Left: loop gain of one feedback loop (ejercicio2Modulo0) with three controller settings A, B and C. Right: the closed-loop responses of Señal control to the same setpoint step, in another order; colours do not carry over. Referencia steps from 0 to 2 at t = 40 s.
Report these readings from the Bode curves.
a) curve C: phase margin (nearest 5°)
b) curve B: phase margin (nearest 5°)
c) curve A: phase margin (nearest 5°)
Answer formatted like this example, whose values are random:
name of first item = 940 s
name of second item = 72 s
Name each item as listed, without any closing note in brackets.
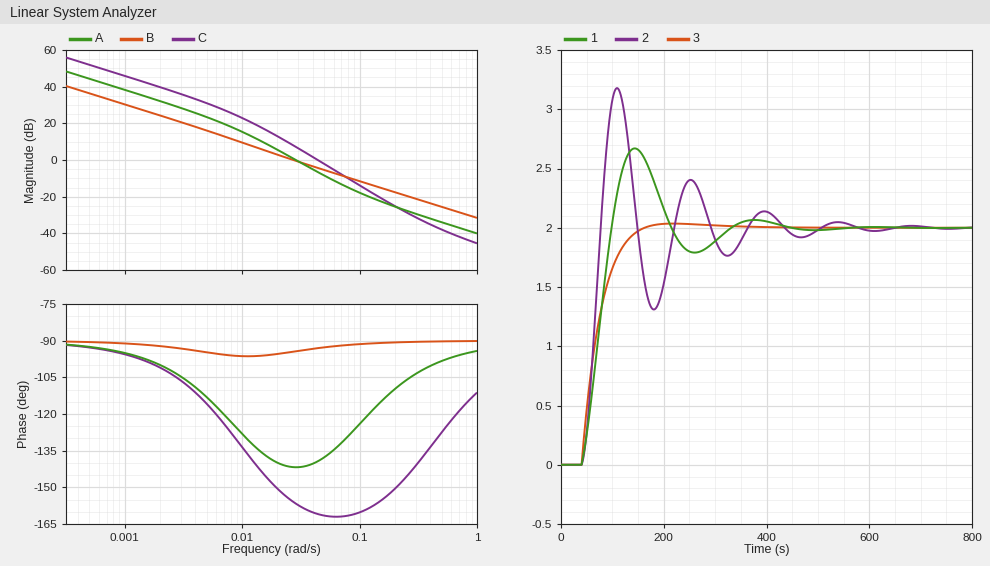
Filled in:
curve C: phase margin = 20°
curve B: phase margin = 85°
curve A: phase margin = 40°
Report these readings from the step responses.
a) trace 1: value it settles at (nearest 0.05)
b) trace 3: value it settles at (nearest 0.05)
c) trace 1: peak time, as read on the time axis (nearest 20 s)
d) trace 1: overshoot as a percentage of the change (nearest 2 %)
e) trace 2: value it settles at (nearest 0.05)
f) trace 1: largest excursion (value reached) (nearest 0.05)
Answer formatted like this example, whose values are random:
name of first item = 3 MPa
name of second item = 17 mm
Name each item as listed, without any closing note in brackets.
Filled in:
trace 1: value it settles at = 2.00
trace 3: value it settles at = 2.00
trace 1: peak time, as read on the time axis = 140 s
trace 1: overshoot as a percentage of the change = 34 %
trace 2: value it settles at = 2.00
trace 1: largest excursion (value reached) = 2.65
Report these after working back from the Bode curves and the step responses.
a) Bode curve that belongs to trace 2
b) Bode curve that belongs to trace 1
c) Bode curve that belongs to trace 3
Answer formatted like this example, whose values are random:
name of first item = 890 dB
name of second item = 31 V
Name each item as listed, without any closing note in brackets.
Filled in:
Bode curve that belongs to trace 2 = C
Bode curve that belongs to trace 1 = A
Bode curve that belongs to trace 3 = B
